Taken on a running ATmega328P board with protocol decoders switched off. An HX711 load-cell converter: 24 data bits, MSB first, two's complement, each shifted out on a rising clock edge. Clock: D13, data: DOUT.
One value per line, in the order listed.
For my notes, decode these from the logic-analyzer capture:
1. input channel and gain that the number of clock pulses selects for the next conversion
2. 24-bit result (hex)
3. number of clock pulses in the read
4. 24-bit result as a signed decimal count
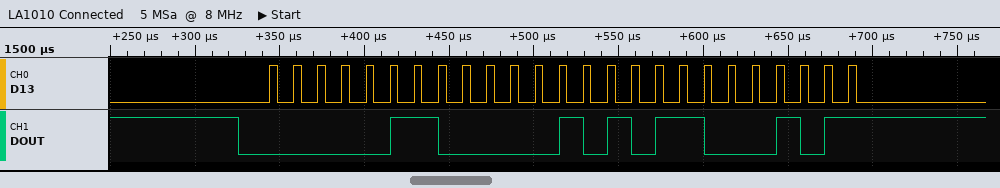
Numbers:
channel A, gain 128
0x060AC5
25
395973
